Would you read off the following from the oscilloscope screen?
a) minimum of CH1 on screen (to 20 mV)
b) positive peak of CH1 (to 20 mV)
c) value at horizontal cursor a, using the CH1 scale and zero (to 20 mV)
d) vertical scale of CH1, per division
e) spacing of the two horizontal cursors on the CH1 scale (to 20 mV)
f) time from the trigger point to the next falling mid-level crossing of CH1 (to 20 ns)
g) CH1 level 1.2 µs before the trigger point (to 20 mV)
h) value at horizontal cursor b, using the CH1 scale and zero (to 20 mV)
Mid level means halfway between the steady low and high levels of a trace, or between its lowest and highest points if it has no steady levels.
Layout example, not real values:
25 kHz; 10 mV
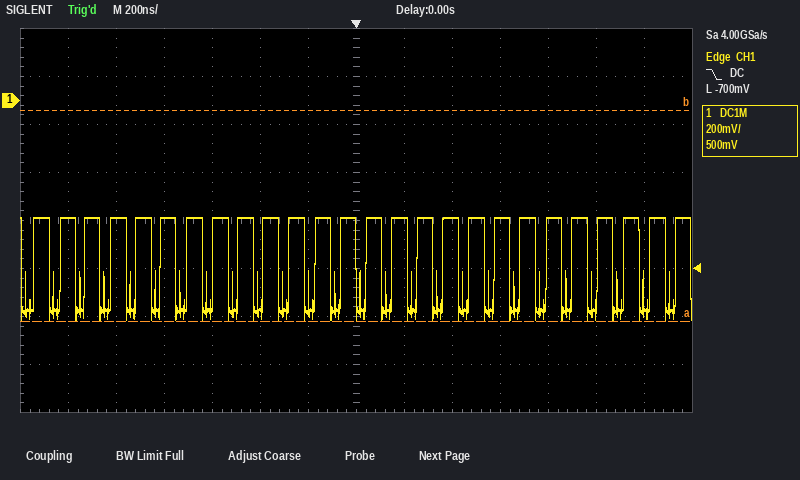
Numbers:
-920 mV; -480 mV; -920 mV; 200 mV; 880 mV; 100 ns; -480 mV; -40 mV
